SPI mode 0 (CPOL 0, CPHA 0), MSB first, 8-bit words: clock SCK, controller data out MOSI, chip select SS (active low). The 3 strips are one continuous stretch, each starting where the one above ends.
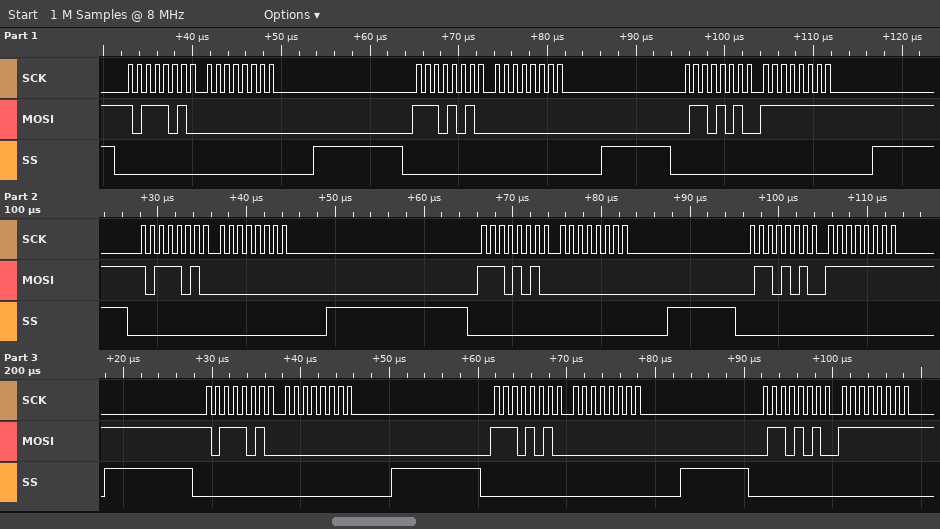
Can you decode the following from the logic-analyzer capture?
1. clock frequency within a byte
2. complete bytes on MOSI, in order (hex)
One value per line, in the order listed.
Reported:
1 MHz
BA 00 EA 00 6A FF BA 00 EA 00 6A FF BA 00 EA 00 6A FF
